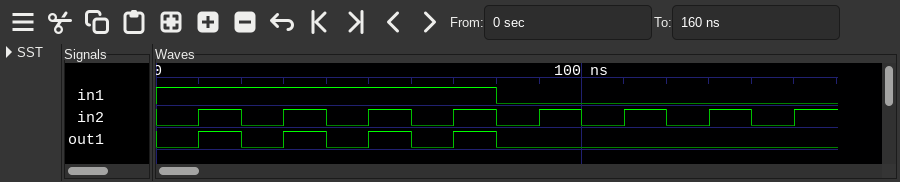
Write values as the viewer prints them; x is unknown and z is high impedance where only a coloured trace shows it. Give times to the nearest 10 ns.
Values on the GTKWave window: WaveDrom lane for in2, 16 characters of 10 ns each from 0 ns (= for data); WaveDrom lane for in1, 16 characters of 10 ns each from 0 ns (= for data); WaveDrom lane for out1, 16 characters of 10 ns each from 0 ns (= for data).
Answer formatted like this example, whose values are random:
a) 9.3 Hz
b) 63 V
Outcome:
a) {name: 'in2', wave: '0101010101010101'}
b) {name: 'in1', wave: '1.......0.......'}
c) {name: 'out1', wave: '010101010.......'}
